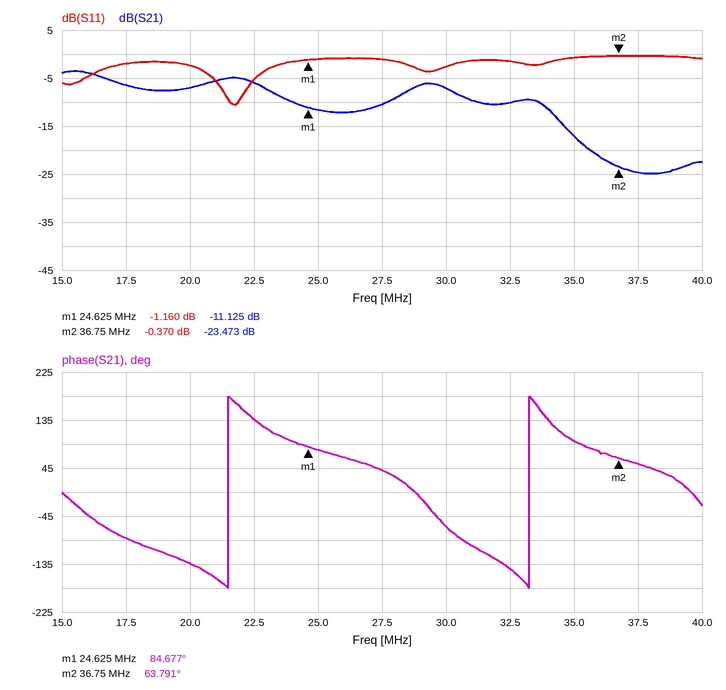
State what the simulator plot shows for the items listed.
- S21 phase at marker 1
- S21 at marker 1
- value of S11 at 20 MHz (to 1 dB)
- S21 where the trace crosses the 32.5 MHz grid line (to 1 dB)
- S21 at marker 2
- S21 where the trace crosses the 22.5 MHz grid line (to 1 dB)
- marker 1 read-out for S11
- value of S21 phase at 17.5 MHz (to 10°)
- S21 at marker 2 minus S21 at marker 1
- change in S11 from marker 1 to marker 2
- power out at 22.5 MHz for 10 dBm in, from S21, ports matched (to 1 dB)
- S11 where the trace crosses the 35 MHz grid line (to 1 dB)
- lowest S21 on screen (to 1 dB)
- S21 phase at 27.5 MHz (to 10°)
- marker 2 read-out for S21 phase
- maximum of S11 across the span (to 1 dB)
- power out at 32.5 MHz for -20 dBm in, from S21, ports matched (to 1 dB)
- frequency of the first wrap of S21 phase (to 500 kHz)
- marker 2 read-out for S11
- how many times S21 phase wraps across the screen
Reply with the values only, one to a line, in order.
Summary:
84.677°
-11.125 dB
-2 dB
-10 dB
-23.473 dB
-6 dB
-1.160 dB
-90°
-12.348 dB
0.790 dB
4 dBm
-1 dB
-25 dB
40°
63.791°
0 dB
-30 dBm
21.5 MHz
-0.370 dB
2
